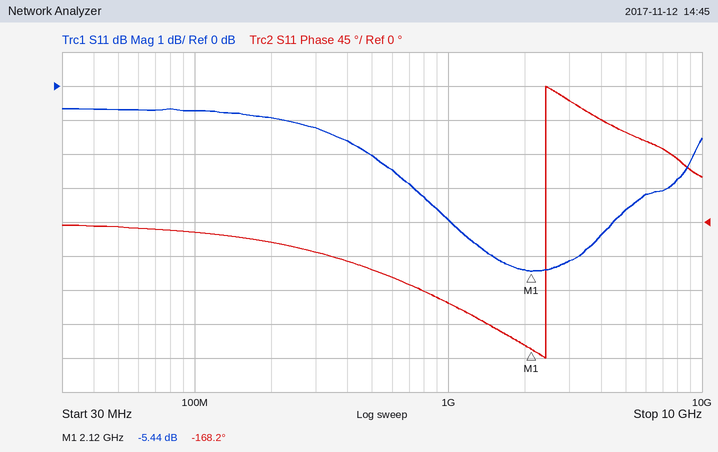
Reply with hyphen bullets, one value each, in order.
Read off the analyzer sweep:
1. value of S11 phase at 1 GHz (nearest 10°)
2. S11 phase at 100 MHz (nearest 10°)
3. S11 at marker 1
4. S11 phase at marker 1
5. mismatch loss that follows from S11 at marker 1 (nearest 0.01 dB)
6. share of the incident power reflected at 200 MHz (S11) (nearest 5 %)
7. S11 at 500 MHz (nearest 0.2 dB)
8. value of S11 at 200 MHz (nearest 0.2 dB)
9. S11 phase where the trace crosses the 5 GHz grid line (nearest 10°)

- -110°
- -10°
- -5.44 dB
- -168.2°
- 1.46 dB
- 80 %
- -2.0 dB
- -1.0 dB
- 120°
